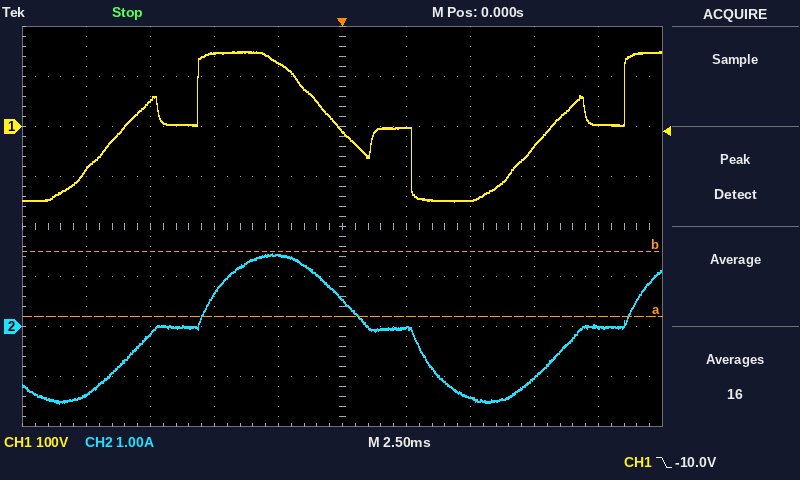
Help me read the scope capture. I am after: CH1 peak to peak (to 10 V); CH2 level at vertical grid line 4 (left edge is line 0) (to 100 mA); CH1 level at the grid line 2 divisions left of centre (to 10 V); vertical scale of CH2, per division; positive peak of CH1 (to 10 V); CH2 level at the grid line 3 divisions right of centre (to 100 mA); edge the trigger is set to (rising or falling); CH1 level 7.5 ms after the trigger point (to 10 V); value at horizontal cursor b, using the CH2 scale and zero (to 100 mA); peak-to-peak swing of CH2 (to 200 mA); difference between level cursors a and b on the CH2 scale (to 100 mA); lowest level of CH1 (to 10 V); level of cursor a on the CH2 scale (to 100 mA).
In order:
300 V
1.4 A
150 V
1 A
150 V
-1.0 A
falling
-40 V
1.5 A
3.0 A
1.3 A
-150 V
200 mA
